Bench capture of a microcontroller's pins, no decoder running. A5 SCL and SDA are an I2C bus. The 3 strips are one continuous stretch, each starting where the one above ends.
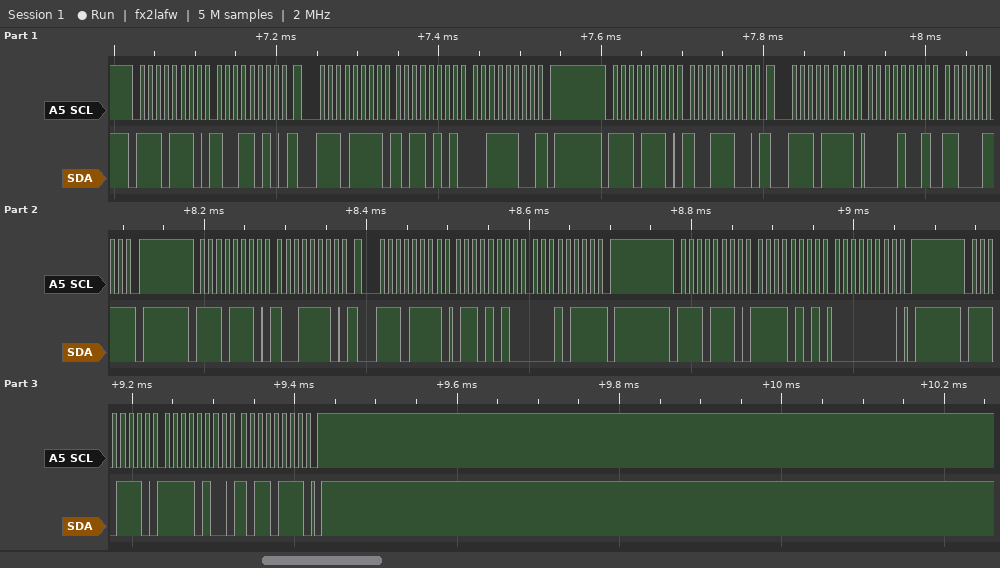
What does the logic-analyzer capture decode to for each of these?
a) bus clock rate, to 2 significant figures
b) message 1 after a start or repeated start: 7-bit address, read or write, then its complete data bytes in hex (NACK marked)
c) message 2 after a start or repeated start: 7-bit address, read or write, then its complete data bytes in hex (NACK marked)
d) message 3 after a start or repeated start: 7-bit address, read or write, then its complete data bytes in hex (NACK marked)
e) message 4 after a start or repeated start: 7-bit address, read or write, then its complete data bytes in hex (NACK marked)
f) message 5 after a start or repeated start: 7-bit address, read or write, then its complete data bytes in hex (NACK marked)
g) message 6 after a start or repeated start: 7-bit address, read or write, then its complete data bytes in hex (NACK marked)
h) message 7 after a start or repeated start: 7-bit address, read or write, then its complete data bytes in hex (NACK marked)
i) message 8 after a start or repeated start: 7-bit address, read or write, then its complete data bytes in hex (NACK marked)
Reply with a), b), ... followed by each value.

a) 100 kHz
b) 0x77 write: 9A
c) 0x77 read: B5 3C NACK
d) 0x77 write: 9C
e) 0x77 read: 09 C7 NACK
f) 0x77 write: 9E
g) 0x77 read: 6A 17 NACK
h) 0x77 write: F5 00
i) 0x77 write: F4 B7
